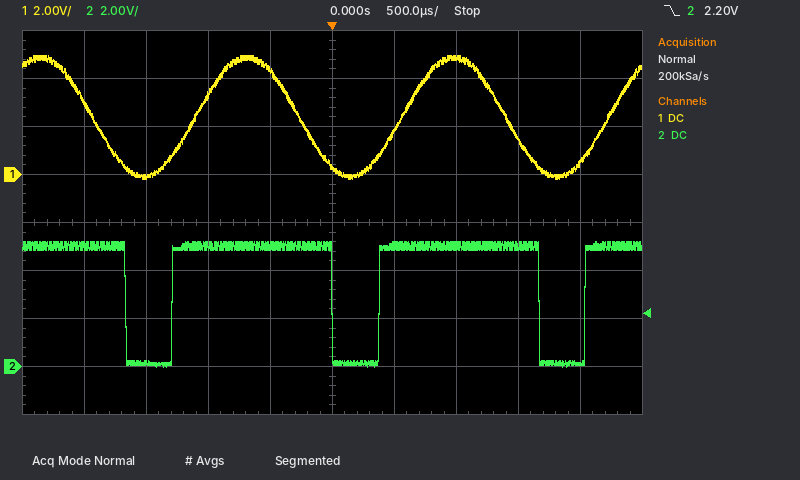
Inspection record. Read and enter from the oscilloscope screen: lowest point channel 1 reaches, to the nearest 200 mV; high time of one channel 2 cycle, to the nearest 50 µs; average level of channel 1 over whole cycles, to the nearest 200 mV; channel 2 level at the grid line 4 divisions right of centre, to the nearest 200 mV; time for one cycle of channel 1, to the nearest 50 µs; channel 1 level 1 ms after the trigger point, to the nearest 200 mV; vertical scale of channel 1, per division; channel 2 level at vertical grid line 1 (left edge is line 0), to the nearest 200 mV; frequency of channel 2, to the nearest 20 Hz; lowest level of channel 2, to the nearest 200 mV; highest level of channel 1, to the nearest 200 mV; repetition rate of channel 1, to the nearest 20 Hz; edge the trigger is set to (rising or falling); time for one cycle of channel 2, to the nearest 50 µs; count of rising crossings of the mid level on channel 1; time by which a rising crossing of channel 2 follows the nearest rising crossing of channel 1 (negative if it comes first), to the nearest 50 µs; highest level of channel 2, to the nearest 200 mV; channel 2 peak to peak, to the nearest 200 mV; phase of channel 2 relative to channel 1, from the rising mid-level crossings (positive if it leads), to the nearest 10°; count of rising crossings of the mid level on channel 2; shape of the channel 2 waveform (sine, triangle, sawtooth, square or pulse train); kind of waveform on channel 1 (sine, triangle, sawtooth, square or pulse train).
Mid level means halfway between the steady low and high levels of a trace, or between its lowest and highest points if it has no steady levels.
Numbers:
-200 mV
1.30 ms
2.4 V
200 mV
1.65 ms
4.8 V
2 V
5.0 V
600 Hz
0.0 V
5.0 V
600 Hz
falling
1.65 ms
3
-200 µs
5.2 V
5.2 V
+40°
3
pulse train
sine
